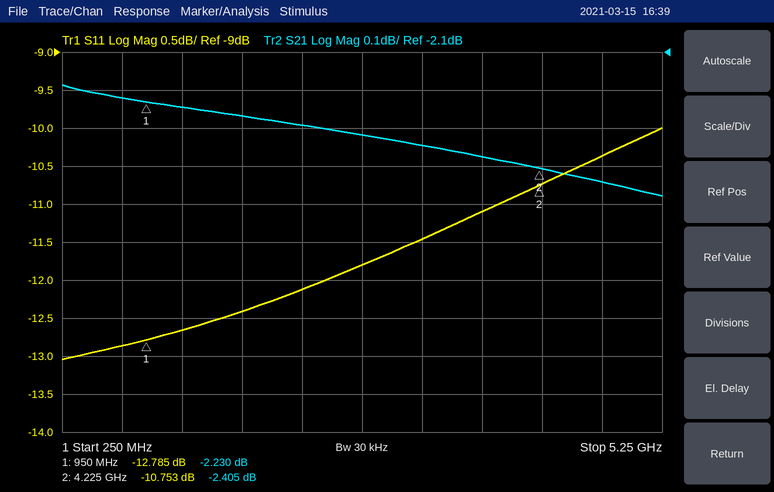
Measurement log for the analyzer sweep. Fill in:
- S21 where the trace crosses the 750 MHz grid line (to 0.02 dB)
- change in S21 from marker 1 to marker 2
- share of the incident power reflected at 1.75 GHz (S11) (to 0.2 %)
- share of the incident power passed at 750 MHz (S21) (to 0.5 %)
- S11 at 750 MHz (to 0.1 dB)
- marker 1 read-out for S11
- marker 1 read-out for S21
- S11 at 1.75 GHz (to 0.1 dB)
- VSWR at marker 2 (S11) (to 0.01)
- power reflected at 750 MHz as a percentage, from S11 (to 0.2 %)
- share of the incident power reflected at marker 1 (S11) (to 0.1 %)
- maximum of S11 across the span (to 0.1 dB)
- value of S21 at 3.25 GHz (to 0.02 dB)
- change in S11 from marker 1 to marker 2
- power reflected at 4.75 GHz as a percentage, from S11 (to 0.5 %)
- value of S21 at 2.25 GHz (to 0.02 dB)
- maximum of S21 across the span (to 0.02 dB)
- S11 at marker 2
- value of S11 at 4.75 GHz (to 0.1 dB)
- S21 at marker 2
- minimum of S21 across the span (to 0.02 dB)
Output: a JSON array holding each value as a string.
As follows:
["-2.22 dB", "-0.175 dB", "5.8 %", "60.0 %", "-12.9 dB", "-12.785 dB", "-2.230 dB", "-12.4 dB", "1.82", "5.2 %", "5.3 %", "-10.0 dB", "-2.34 dB", "2.032 dB", "9.0 %", "-2.30 dB", "-2.18 dB", "-10.753 dB", "-10.4 dB", "-2.405 dB", "-2.48 dB"]
